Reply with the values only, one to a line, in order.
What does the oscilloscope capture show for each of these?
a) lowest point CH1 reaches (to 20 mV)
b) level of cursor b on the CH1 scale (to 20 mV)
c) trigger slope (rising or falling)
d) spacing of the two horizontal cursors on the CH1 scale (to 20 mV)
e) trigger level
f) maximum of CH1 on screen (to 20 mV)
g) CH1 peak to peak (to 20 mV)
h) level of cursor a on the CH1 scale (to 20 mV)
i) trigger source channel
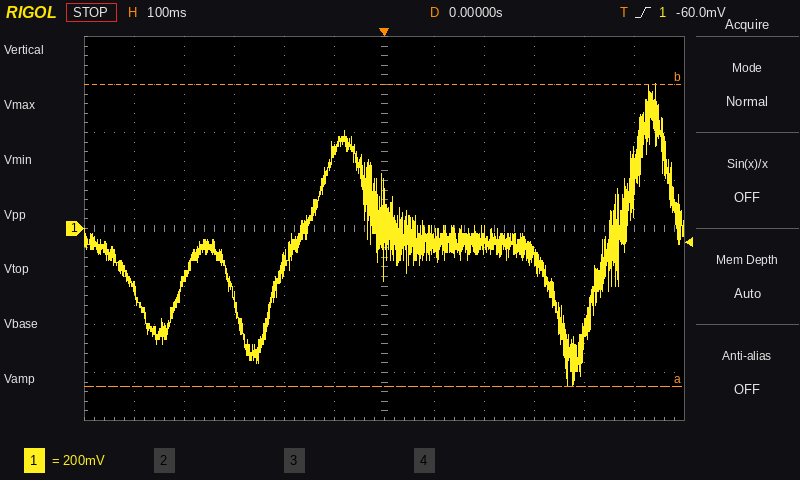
-660 mV
600 mV
rising
1.26 V
-60.0 mV
600 mV
1.26 V
-660 mV
CH1
